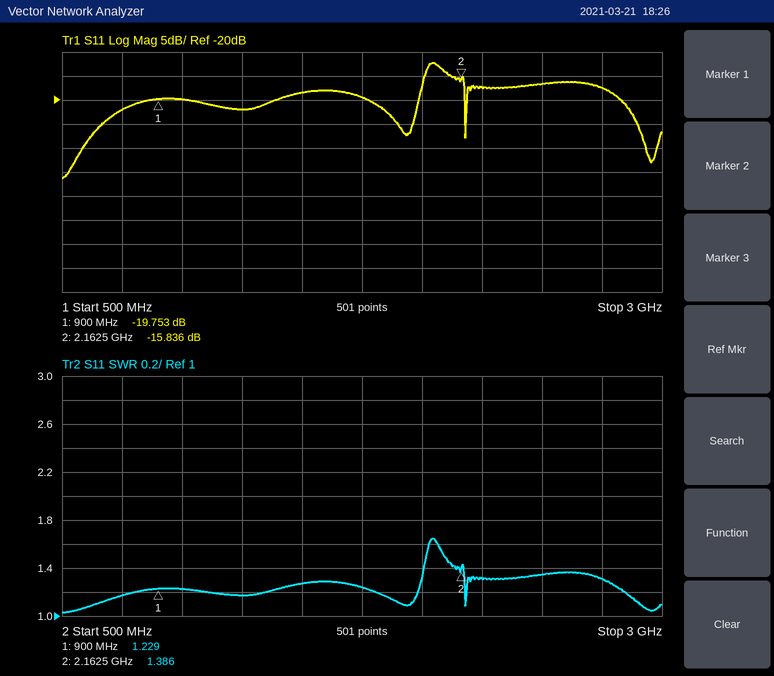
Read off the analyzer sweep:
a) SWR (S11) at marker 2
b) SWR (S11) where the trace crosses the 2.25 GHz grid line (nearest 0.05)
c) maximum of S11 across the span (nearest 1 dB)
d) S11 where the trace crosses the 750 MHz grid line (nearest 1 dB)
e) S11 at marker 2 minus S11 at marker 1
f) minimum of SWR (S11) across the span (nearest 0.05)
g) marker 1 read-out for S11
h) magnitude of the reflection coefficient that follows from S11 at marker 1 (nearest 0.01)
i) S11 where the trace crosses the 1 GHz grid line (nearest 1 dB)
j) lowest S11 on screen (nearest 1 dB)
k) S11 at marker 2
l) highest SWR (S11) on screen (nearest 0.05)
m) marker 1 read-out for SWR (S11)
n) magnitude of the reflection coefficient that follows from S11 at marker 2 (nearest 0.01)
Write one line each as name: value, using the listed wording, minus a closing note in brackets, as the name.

SWR (S11) at marker 2: 1.386
SWR (S11) where the trace crosses the 2.25 GHz grid line: 1.30
maximum of S11 across the span: -12 dB
S11 where the trace crosses the 750 MHz grid line: -22 dB
S11 at marker 2 minus S11 at marker 1: 3.917 dB
minimum of SWR (S11) across the span: 1.05
marker 1 read-out for S11: -19.753 dB
magnitude of the reflection coefficient that follows from S11 at marker 1: 0.10
S11 where the trace crosses the 1 GHz grid line: -20 dB
lowest S11 on screen: -36 dB
S11 at marker 2: -15.836 dB
highest SWR (S11) on screen: 1.65
marker 1 read-out for SWR: 1.229
magnitude of the reflection coefficient that follows from S11 at marker 2: 0.16
